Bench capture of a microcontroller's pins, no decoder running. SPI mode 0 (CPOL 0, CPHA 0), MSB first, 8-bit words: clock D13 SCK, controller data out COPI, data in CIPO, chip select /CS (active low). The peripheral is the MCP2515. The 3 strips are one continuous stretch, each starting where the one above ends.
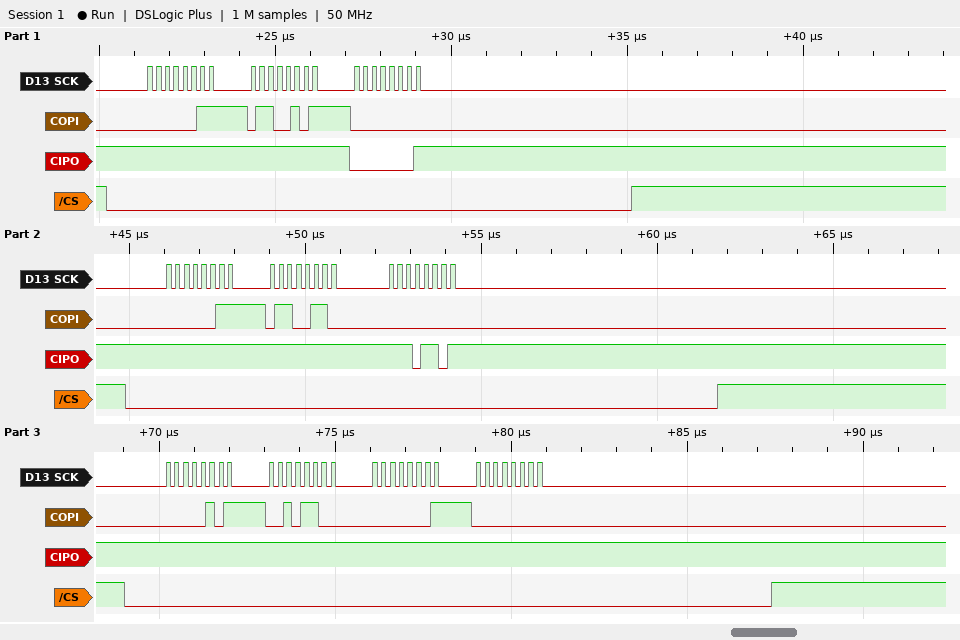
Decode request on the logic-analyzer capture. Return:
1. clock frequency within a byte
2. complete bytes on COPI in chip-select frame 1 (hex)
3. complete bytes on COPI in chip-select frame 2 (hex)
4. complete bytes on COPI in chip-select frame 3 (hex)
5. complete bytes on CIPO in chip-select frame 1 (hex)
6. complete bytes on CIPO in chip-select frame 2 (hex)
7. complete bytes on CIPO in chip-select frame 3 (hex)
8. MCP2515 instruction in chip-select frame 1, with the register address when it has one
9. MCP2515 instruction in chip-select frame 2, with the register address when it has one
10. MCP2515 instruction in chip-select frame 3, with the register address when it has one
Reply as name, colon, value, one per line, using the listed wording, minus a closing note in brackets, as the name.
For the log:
clock frequency within a byte: 4 MHz
complete bytes on COPI in chip-select frame 1: 03 65 00
complete bytes on COPI in chip-select frame 2: 03 66 00
complete bytes on COPI in chip-select frame 3: 05 2C 01 00
complete bytes on CIPO in chip-select frame 1: FF FF 01
complete bytes on CIPO in chip-select frame 2: FF FF ED
complete bytes on CIPO in chip-select frame 3: FF FF FF FF
MCP2515 instruction in chip-select frame 1, with the register address when it has one: READ 0x65
MCP2515 instruction in chip-select frame 2, with the register address when it has one: READ 0x66
MCP2515 instruction in chip-select frame 3, with the register address when it has one: BIT MODIFY 0x2C
